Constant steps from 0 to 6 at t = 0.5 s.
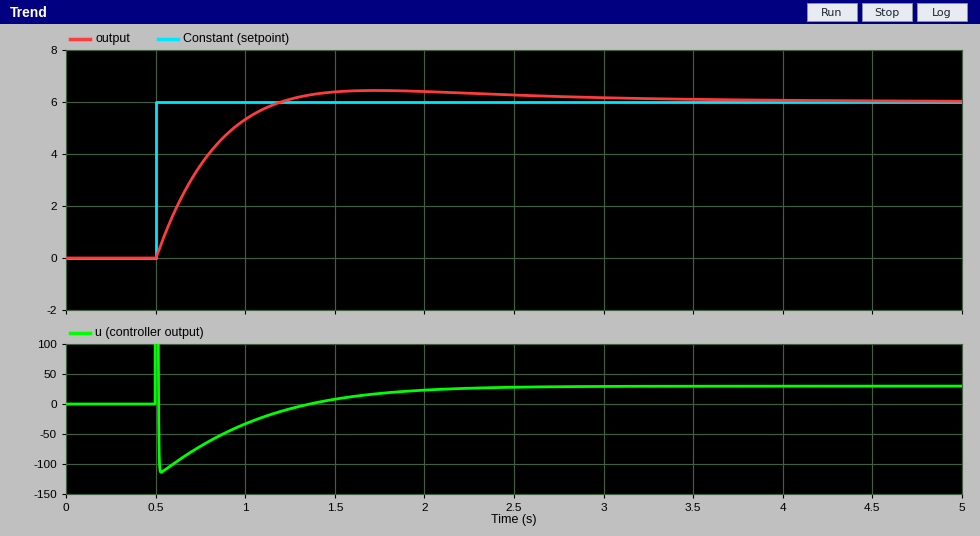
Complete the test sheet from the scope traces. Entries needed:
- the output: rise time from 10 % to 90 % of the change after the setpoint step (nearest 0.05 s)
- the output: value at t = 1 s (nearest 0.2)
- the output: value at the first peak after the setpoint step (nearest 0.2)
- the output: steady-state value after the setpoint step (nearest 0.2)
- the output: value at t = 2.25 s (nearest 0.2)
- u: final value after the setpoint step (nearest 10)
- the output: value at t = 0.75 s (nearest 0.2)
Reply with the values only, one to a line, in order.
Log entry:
0.50 s
5.4
6.4
6.0
6.4
30
3.6
